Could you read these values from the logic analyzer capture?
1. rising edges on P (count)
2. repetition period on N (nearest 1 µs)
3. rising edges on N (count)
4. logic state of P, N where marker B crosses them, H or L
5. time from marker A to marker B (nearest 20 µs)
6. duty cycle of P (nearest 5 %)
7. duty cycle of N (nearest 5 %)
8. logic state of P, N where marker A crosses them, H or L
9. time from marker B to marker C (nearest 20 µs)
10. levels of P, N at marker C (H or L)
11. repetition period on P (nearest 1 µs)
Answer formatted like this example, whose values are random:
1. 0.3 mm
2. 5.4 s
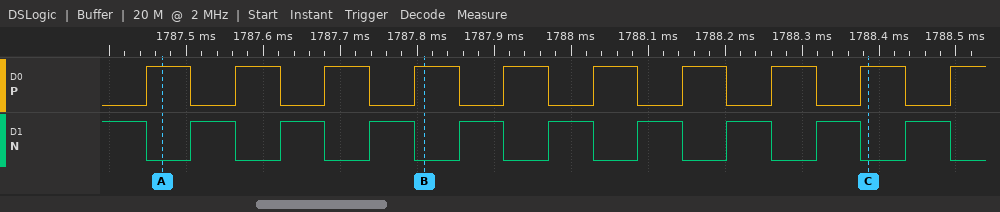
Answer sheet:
1. 10
2. 116 µs
3. 9
4. P=H, N=L
5. 340 µs
6. 50 %
7. 50 %
8. P=H, N=L
9. 580 µs
10. P=H, N=L
11. 116 µs
